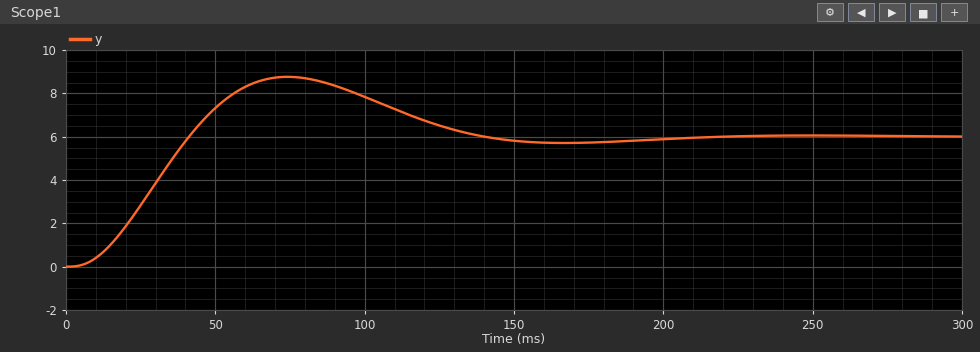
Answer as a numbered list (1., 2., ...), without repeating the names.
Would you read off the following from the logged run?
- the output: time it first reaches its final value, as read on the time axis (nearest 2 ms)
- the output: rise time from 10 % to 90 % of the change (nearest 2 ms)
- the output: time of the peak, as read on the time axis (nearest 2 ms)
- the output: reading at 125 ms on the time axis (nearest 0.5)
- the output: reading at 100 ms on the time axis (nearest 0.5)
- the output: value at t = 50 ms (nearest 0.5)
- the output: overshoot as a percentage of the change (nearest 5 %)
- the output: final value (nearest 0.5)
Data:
1. 42 ms
2. 26 ms
3. 74 ms
4. 6.5
5. 8.0
6. 7.5
7. 45 %
8. 6.0
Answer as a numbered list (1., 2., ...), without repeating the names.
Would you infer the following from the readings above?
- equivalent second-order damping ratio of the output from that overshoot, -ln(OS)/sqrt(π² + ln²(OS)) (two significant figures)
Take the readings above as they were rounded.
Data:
1. 0.25
